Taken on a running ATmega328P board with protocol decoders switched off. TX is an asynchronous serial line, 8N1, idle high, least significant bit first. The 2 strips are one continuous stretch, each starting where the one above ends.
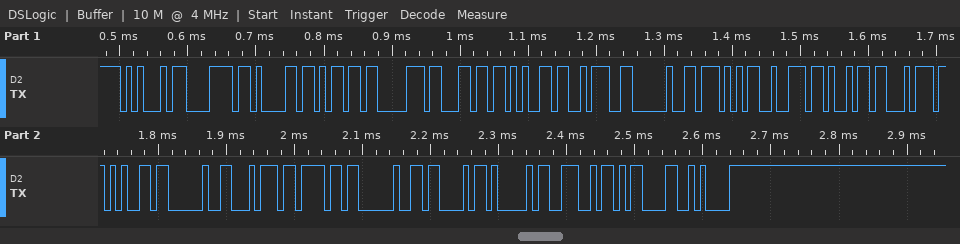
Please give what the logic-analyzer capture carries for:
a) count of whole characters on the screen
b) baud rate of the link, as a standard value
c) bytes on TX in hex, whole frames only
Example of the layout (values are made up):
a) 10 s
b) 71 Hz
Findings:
a) 23
b) 115200 baud
c) 45 78 61 6D 70 6C 65 3A 20 57 72 69 74 65 20 74 6F 20 43 41 4E 0D 0A
